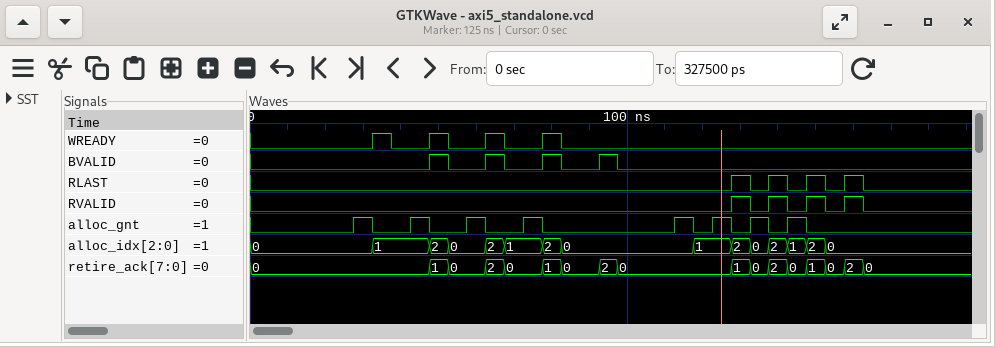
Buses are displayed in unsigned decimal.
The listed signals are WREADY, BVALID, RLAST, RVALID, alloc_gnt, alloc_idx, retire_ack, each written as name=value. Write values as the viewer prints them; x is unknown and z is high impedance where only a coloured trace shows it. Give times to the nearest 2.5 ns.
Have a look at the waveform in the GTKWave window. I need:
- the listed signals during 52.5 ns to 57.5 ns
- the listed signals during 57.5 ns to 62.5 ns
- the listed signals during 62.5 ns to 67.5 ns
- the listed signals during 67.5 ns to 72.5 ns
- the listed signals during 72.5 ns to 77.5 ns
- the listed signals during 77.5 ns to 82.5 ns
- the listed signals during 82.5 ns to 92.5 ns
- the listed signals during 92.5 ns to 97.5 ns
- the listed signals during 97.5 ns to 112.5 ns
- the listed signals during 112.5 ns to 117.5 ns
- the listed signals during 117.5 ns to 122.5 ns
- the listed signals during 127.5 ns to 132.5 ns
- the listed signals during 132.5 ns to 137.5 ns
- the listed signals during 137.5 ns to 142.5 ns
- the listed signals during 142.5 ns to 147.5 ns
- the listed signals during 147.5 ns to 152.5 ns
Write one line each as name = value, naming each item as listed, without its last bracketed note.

the listed signals during 52.5 ns to 57.5 ns = WREADY=0, BVALID=0, RLAST=0, RVALID=0, alloc_gnt=0, alloc_idx=0, retire_ack=0
the listed signals during 57.5 ns to 62.5 ns = WREADY=0, BVALID=0, RLAST=0, RVALID=0, alloc_gnt=1, alloc_idx=0, retire_ack=0
the listed signals during 62.5 ns to 67.5 ns = WREADY=1, BVALID=1, RLAST=0, RVALID=0, alloc_gnt=0, alloc_idx=2, retire_ack=2
the listed signals during 67.5 ns to 72.5 ns = WREADY=0, BVALID=0, RLAST=0, RVALID=0, alloc_gnt=0, alloc_idx=1, retire_ack=0
the listed signals during 72.5 ns to 77.5 ns = WREADY=0, BVALID=0, RLAST=0, RVALID=0, alloc_gnt=1, alloc_idx=1, retire_ack=0
the listed signals during 77.5 ns to 82.5 ns = WREADY=1, BVALID=1, RLAST=0, RVALID=0, alloc_gnt=0, alloc_idx=2, retire_ack=1
the listed signals during 82.5 ns to 92.5 ns = WREADY=0, BVALID=0, RLAST=0, RVALID=0, alloc_gnt=0, alloc_idx=0, retire_ack=0
the listed signals during 92.5 ns to 97.5 ns = WREADY=0, BVALID=1, RLAST=0, RVALID=0, alloc_gnt=0, alloc_idx=0, retire_ack=2
the listed signals during 97.5 ns to 112.5 ns = WREADY=0, BVALID=0, RLAST=0, RVALID=0, alloc_gnt=0, alloc_idx=0, retire_ack=0
the listed signals during 112.5 ns to 117.5 ns = WREADY=0, BVALID=0, RLAST=0, RVALID=0, alloc_gnt=1, alloc_idx=0, retire_ack=0
the listed signals during 117.5 ns to 122.5 ns = WREADY=0, BVALID=0, RLAST=0, RVALID=0, alloc_gnt=0, alloc_idx=1, retire_ack=0
the listed signals during 127.5 ns to 132.5 ns = WREADY=0, BVALID=0, RLAST=1, RVALID=1, alloc_gnt=0, alloc_idx=2, retire_ack=1
the listed signals during 132.5 ns to 137.5 ns = WREADY=0, BVALID=0, RLAST=0, RVALID=0, alloc_gnt=1, alloc_idx=0, retire_ack=0
the listed signals during 137.5 ns to 142.5 ns = WREADY=0, BVALID=0, RLAST=1, RVALID=1, alloc_gnt=0, alloc_idx=2, retire_ack=2
the listed signals during 142.5 ns to 147.5 ns = WREADY=0, BVALID=0, RLAST=0, RVALID=0, alloc_gnt=1, alloc_idx=1, retire_ack=0
the listed signals during 147.5 ns to 152.5 ns = WREADY=0, BVALID=0, RLAST=1, RVALID=1, alloc_gnt=0, alloc_idx=2, retire_ack=1
